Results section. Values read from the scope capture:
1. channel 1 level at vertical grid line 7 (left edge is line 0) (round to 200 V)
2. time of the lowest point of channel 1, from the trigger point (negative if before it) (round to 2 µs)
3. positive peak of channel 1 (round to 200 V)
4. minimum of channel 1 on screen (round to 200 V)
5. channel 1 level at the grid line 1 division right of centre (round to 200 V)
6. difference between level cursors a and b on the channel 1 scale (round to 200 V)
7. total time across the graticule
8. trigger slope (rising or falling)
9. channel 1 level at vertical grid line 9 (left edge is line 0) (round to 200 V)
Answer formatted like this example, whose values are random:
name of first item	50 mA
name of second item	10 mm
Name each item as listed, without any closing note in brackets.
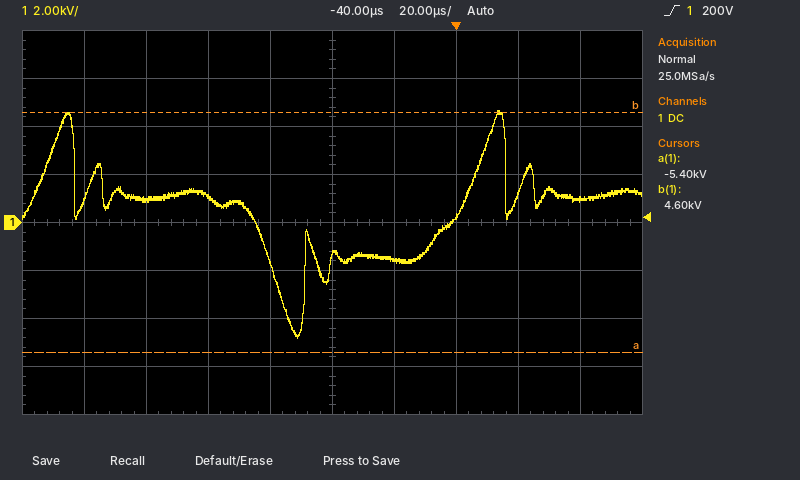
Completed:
channel 1 level at vertical grid line 7 (left edge is line 0)	200 V
time of the lowest point of channel 1, from the trigger point (negative if before it)	-52 µs
positive peak of channel 1	4.6 kV
minimum of channel 1 on screen	-4.8 kV
channel 1 level at the grid line 1 division right of centre	-1.6 kV
difference between level cursors a and b on the channel 1 scale	10.0 kV
total time across the graticule	200 µs
trigger slope	rising
channel 1 level at vertical grid line 9 (left edge is line 0)	1.0 kV
